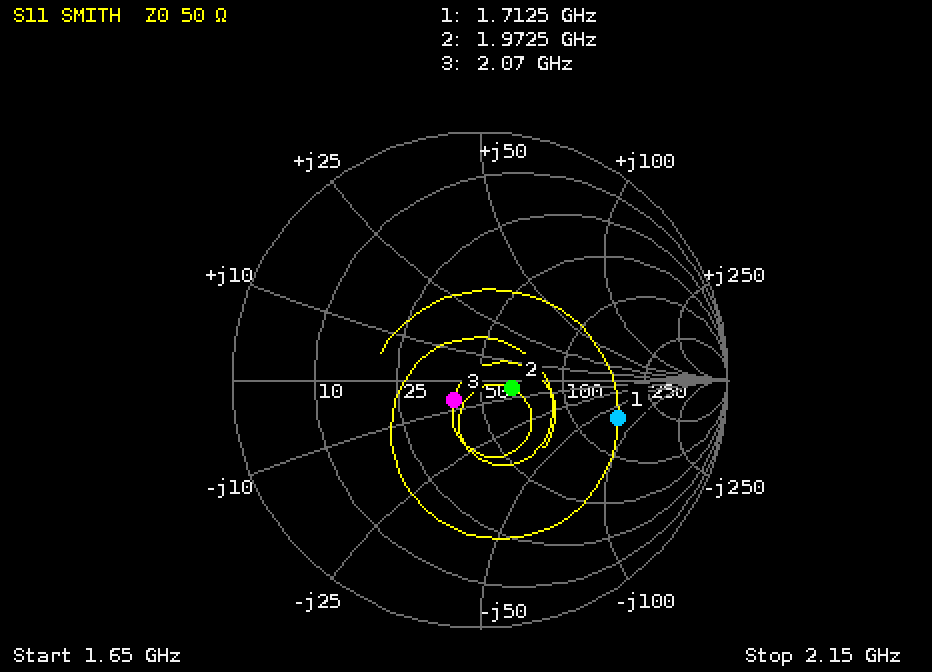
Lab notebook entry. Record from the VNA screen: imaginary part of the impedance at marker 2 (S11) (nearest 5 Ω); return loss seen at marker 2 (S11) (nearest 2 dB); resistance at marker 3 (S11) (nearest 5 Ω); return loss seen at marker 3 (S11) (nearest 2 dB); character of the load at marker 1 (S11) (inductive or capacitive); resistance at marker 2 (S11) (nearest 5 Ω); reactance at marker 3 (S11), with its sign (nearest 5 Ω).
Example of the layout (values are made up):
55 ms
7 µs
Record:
-5 Ω
18 dB
40 Ω
18 dB
capacitive
65 Ω
-5 Ω
